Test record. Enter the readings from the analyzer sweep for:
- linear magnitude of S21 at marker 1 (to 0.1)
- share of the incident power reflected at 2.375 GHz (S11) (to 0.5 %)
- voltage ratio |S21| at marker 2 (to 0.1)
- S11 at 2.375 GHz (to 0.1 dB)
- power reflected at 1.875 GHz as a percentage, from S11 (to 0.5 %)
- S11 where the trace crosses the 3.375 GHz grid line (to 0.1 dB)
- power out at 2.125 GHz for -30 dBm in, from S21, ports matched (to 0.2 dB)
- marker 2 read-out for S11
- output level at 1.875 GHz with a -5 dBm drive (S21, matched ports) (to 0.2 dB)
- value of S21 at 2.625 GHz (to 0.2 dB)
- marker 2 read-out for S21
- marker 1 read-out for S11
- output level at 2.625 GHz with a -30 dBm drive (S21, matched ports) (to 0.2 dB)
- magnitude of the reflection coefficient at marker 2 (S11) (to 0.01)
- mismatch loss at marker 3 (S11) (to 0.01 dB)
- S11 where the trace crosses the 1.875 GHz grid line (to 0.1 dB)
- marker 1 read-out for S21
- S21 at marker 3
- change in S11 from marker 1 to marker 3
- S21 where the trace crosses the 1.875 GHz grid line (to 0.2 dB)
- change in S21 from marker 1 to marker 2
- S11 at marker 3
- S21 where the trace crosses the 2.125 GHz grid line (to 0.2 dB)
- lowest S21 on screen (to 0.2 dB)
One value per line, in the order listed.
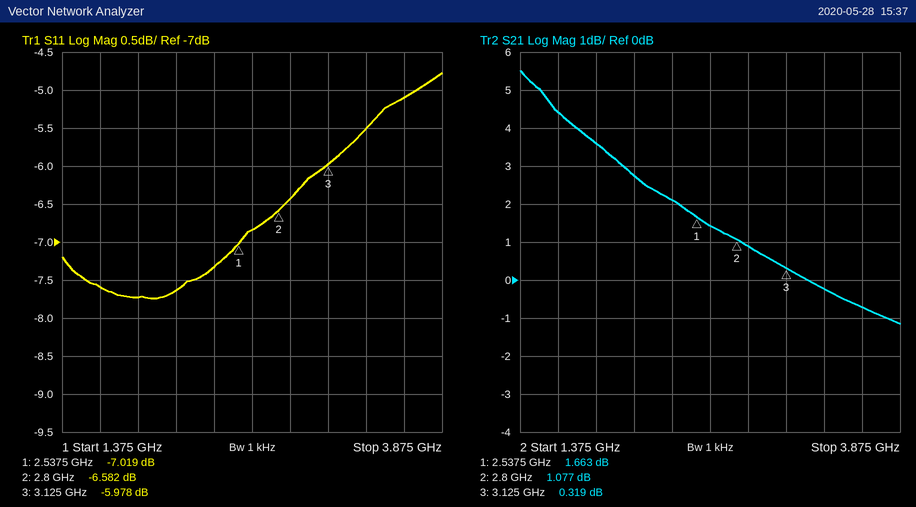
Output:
1.2
18.5 %
1.1
-7.3 dB
17.0 %
-5.5 dB
-27.2 dBm
-6.582 dB
-1.4 dBm
1.4 dB
1.077 dB
-7.019 dB
-28.6 dBm
0.47
1.26 dB
-7.7 dB
1.663 dB
0.319 dB
1.041 dB
3.6 dB
-0.586 dB
-5.978 dB
2.8 dB
-1.2 dB
